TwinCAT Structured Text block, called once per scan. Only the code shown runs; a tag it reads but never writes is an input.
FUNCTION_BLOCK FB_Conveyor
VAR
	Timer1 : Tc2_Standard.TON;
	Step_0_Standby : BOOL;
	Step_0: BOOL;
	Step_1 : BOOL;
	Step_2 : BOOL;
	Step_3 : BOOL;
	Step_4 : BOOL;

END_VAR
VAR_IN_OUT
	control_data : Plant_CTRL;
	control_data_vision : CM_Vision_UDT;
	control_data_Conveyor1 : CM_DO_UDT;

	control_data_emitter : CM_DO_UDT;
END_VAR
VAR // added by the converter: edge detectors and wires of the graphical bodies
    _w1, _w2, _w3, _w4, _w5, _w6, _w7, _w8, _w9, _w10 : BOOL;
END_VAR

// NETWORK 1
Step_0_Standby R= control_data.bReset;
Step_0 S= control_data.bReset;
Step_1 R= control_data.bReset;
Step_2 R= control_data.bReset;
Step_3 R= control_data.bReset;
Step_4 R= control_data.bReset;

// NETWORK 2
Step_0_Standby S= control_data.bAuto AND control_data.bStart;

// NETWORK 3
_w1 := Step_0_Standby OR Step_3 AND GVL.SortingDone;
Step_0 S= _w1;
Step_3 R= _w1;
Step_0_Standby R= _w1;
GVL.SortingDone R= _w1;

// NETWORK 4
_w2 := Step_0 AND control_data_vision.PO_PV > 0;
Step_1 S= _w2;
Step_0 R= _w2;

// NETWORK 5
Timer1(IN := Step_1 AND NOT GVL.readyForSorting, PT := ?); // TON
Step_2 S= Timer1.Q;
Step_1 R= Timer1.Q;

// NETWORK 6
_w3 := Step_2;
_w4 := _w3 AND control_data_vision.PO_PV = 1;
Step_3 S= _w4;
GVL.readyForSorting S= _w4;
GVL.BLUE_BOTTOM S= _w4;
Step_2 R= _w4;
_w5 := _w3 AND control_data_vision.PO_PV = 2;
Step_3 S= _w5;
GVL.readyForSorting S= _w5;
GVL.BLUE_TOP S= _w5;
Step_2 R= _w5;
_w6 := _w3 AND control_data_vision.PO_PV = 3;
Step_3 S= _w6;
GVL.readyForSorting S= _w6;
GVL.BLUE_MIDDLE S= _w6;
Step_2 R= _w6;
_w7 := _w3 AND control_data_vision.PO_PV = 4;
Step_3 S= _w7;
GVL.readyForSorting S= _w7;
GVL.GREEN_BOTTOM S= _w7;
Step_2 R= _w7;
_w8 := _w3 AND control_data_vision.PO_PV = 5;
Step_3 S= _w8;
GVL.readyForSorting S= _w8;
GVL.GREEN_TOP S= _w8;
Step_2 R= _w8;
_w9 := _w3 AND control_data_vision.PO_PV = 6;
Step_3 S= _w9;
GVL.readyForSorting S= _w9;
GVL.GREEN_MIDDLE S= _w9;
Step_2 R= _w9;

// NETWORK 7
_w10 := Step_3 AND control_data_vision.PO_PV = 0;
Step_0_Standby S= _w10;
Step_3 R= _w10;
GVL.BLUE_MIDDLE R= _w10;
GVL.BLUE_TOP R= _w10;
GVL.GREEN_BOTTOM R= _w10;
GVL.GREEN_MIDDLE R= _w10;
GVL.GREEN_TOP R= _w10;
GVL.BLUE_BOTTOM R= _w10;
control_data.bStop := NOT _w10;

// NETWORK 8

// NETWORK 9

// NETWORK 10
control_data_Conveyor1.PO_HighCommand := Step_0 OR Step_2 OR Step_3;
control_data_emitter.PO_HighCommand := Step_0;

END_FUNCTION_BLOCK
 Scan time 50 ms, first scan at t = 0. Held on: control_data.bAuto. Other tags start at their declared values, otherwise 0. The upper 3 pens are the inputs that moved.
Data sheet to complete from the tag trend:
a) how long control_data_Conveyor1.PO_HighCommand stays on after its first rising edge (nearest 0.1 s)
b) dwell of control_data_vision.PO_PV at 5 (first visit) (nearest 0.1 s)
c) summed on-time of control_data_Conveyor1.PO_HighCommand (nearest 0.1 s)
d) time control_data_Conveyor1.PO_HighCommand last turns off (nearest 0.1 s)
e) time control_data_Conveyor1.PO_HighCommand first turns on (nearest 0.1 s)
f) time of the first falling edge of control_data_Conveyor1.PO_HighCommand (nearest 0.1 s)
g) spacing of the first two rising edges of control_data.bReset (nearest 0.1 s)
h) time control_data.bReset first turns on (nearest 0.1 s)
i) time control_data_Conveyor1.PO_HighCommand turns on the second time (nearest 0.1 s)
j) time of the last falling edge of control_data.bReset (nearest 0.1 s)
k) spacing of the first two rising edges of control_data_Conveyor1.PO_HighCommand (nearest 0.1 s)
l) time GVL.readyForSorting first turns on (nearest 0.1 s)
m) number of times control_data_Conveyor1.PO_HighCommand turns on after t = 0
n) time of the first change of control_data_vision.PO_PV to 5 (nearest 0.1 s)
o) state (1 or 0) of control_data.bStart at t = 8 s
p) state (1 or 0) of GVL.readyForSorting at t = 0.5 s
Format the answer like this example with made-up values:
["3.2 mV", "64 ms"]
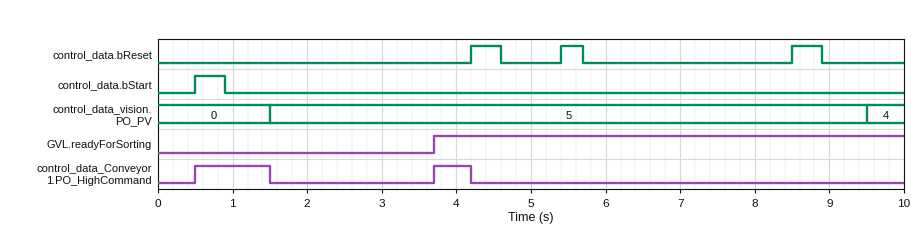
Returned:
["1.0 s", "8.0 s", "1.5 s", "4.2 s", "0.5 s", "1.5 s", "1.2 s", "4.2 s", "3.7 s", "8.9 s", "3.2 s", "3.7 s", "2", "1.5 s", "0", "0"]
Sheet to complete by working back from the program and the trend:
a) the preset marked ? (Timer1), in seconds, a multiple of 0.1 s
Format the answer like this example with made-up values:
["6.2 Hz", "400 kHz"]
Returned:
["2.2 s"]
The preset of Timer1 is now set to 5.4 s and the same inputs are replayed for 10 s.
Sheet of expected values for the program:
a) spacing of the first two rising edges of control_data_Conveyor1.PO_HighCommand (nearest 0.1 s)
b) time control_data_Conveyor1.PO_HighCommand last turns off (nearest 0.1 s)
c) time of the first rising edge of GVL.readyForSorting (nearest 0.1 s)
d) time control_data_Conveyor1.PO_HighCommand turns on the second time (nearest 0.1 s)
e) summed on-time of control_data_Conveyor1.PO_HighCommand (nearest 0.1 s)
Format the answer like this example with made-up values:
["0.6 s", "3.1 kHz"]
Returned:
["6.4 s", "8.5 s", "6.9 s", "6.9 s", "2.6 s"]
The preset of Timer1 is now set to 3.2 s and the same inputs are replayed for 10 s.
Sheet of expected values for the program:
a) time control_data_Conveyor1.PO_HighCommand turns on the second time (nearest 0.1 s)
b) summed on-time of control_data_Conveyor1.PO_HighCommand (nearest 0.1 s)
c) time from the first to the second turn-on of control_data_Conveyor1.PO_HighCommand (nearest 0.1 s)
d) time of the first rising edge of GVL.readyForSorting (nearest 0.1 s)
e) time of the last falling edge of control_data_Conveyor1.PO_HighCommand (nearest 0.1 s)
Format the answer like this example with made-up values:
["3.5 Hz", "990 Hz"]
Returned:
["4.7 s", "1.7 s", "4.2 s", "4.7 s", "5.4 s"]
